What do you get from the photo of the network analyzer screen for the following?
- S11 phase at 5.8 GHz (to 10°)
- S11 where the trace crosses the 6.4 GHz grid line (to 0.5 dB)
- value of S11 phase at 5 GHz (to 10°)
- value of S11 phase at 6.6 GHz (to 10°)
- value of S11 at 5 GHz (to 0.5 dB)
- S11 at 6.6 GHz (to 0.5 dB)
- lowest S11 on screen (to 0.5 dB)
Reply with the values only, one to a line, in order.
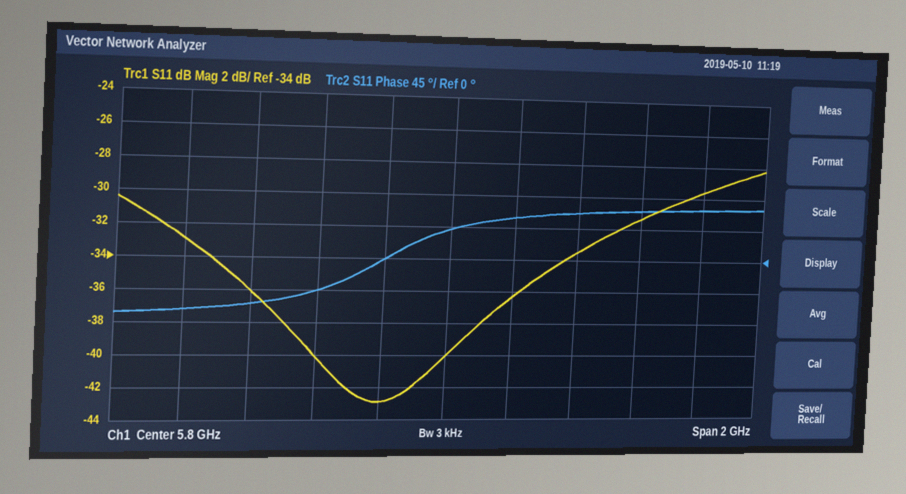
40°
-31.5 dB
-70°
70°
-33.0 dB
-29.5 dB
-43.0 dB
